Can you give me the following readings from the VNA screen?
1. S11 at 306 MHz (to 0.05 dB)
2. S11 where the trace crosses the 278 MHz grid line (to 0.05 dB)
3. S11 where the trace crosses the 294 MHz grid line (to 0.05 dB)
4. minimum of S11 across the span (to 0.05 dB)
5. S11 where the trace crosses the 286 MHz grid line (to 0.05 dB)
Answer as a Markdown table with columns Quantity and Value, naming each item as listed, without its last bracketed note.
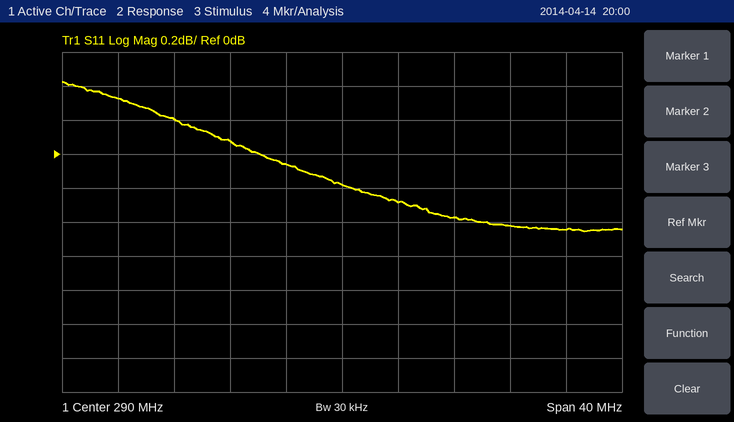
| Quantity | Value |
|---|---|
| S11 at 306 MHz | -0.45 dB |
| S11 where the trace crosses the 278 MHz grid line | 0.20 dB |
| S11 where the trace crosses the 294 MHz grid line | -0.30 dB |
| minimum of S11 across the span | -0.45 dB |
| S11 where the trace crosses the 286 MHz grid line | -0.05 dB |
